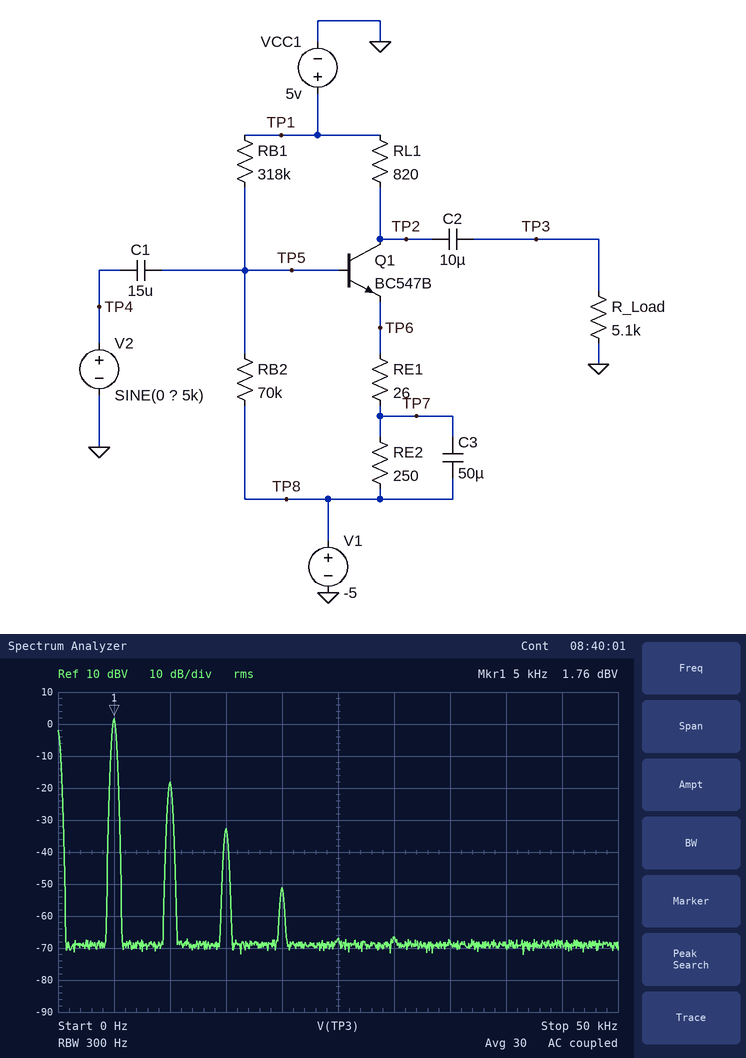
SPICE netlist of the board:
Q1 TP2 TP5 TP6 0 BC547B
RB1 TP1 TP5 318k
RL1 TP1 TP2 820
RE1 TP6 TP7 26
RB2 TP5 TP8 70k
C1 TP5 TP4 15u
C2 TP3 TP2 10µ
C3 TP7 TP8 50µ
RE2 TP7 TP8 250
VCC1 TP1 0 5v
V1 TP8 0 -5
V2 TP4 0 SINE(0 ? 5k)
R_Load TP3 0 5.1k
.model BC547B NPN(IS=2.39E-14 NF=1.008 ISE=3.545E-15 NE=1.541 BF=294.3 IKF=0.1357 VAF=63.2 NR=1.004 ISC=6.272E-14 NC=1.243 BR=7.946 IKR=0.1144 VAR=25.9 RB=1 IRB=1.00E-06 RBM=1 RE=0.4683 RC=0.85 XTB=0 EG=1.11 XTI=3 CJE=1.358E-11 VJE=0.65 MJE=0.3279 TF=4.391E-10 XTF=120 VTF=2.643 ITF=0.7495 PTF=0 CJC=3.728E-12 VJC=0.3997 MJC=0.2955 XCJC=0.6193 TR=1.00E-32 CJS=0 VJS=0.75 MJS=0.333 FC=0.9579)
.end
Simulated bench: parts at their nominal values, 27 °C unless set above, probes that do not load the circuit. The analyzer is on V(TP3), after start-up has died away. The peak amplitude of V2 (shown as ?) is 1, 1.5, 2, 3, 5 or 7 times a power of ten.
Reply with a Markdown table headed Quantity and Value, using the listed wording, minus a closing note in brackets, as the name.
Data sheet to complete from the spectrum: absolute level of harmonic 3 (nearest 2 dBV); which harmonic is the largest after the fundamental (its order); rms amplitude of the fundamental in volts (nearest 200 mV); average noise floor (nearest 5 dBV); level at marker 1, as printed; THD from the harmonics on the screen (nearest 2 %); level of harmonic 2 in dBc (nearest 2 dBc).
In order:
| Quantity | Value |
|---|---|
| absolute level of harmonic 3 | -32 dBV |
| which harmonic is the largest after the fundamental | 2 |
| rms amplitude of the fundamental in volts | 1.2 V |
| average noise floor | -70 dBV |
| level at marker 1, as printed | 1.76 dBV |
| THD from the harmonics on the screen | 10 % |
| level of harmonic 2 in dBc | -20 dBc |
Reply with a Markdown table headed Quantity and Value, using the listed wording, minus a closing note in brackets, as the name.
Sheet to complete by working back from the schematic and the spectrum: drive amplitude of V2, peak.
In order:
| Quantity | Value |
|---|---|
| drive amplitude of V2, peak | 100 mV |
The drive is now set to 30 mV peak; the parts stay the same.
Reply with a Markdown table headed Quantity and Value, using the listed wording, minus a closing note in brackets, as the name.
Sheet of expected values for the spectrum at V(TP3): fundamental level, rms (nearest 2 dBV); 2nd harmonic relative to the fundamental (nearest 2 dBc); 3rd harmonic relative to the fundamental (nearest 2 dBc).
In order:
| Quantity | Value |
|---|---|
| fundamental level, rms | -8 dBV |
| 2nd harmonic relative to the fundamental | -32 dBc |
| 3rd harmonic relative to the fundamental | -56 dBc |
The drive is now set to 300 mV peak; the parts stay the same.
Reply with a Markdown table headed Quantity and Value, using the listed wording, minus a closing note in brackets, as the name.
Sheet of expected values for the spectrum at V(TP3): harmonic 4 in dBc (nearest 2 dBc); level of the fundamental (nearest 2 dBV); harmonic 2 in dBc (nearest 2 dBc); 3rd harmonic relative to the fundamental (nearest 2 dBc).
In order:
| Quantity | Value |
|---|---|
| harmonic 4 in dBc | -24 dBc |
| level of the fundamental | 6 dBV |
| harmonic 2 in dBc | -8 dBc |
| 3rd harmonic relative to the fundamental | -32 dBc |
